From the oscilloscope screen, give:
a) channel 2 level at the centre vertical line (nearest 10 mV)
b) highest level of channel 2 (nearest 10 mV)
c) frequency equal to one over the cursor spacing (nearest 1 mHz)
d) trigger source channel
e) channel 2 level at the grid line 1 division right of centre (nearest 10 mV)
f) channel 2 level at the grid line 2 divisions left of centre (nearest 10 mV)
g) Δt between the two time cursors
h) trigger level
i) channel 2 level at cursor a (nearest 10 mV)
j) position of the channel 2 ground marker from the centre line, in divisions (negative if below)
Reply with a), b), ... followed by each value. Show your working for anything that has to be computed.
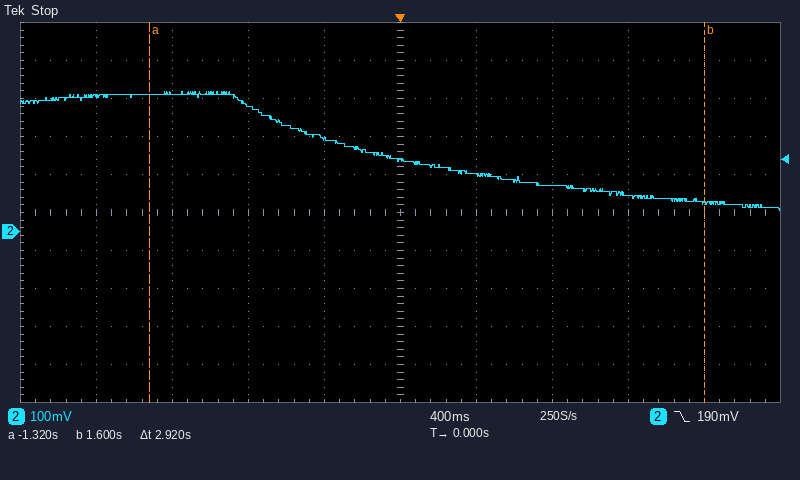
a) 190 mV
b) 370 mV
c) 1 / 2.92 s ≈ 342 mHz
d) channel 2
e) 150 mV
f) 330 mV
g) 2.92 s
h) 190 mV
i) 360 mV
j) -0.5 div
